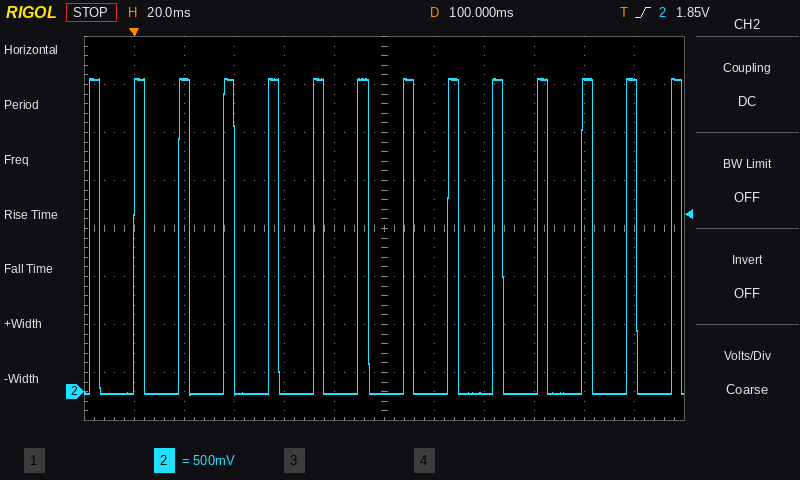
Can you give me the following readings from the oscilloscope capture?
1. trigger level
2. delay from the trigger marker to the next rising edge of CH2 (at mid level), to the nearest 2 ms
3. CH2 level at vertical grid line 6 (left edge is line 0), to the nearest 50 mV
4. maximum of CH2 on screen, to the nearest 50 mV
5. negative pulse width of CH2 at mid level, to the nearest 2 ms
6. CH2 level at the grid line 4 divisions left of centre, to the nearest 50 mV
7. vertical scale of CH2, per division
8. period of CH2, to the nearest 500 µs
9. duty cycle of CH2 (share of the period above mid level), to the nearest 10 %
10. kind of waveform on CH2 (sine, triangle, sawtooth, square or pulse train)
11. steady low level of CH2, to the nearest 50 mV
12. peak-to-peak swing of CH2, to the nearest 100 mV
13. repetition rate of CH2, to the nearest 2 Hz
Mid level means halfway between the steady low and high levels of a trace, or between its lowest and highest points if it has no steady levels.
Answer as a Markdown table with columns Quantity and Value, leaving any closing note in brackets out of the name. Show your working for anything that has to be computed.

| Quantity | Value |
|---|---|
| trigger level | 1.85 V |
| delay from the trigger marker to the next rising edge of CH2 (at mid level), to the nearest 2 ms | 18 ms |
| CH2 level at vertical grid line 6 (left edge is line 0), to the nearest 50 mV | 0 mV |
| maximum of CH2 on screen, to the nearest 50 mV | 3.25 V |
| negative pulse width of CH2 at mid level, to the nearest 2 ms | 14 ms |
| CH2 level at the grid line 4 divisions left of centre, to the nearest 50 mV | 3.25 V |
| vertical scale of CH2, per division | 500 mV |
| period of CH2, to the nearest 500 µs | 18.0 ms |
| duty cycle of CH2 (share of the period above mid level), to the nearest 10 % | 20 % |
| kind of waveform on CH2 | pulse train |
| steady low level of CH2, to the nearest 50 mV | 0 mV |
| peak-to-peak swing of CH2, to the nearest 100 mV | 3.30 V |
| repetition rate of CH2, to the nearest 2 Hz | 1 / 18.0 ms ≈ 56 Hz |
